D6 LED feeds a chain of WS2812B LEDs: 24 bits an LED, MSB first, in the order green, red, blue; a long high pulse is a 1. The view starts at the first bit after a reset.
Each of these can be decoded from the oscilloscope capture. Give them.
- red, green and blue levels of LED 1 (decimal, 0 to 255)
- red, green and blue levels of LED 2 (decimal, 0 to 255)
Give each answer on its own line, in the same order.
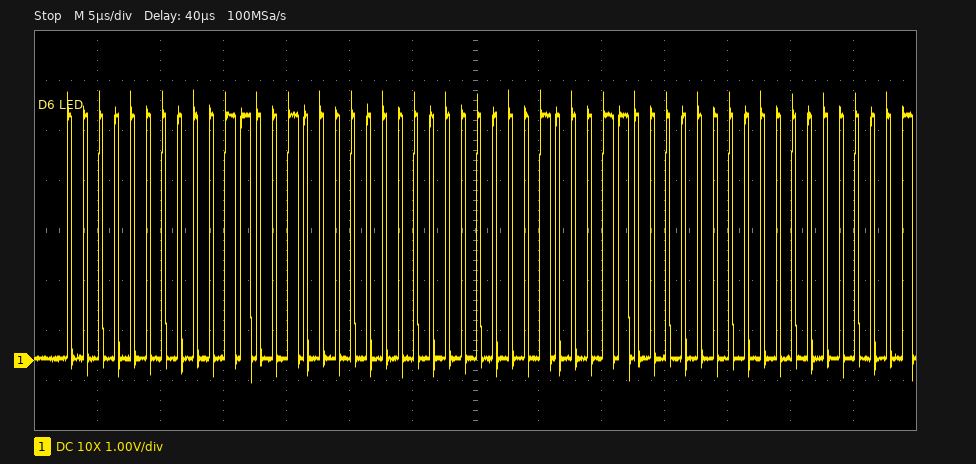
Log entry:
50, 0, 0
48, 2, 0
